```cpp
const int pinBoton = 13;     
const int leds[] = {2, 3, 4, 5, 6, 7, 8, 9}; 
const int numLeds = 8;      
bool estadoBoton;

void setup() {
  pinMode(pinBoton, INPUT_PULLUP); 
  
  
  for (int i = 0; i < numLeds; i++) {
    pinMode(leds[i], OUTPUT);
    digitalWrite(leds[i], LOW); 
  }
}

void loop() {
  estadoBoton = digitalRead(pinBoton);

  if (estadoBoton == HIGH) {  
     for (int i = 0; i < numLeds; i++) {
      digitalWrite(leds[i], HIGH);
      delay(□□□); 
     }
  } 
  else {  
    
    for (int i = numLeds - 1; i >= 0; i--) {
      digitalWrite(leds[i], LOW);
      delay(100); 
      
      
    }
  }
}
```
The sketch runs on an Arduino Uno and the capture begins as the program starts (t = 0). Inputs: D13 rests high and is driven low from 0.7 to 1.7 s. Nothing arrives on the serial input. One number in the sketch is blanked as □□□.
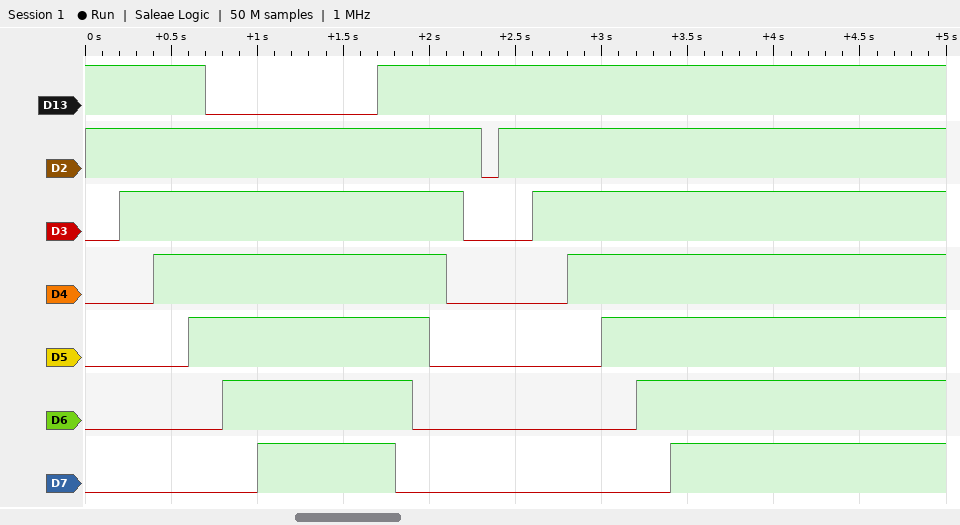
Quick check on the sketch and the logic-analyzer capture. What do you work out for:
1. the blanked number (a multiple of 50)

200
